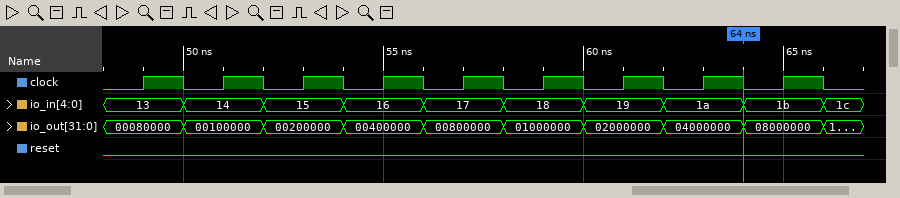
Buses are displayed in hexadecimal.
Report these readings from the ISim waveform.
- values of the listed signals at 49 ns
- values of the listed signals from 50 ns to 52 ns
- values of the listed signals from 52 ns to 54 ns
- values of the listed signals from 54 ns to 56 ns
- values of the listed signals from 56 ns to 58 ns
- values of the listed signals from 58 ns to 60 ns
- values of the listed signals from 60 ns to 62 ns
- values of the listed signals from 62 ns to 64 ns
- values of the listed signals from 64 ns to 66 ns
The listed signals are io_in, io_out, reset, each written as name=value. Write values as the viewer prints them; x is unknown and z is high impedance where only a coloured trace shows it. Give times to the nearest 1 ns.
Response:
io_in=13, io_out=00080000, reset=0
io_in=14, io_out=00100000, reset=0
io_in=15, io_out=00200000, reset=0
io_in=16, io_out=00400000, reset=0
io_in=17, io_out=00800000, reset=0
io_in=18, io_out=01000000, reset=0
io_in=19, io_out=02000000, reset=0
io_in=1a, io_out=04000000, reset=0
io_in=1b, io_out=08000000, reset=0
